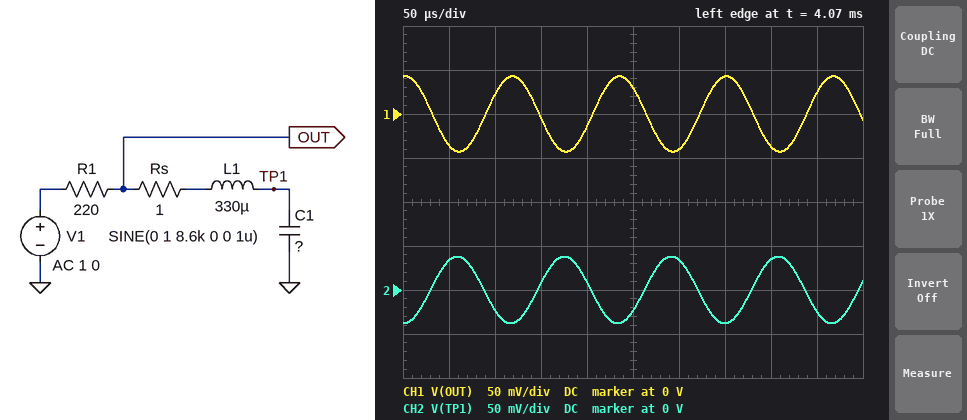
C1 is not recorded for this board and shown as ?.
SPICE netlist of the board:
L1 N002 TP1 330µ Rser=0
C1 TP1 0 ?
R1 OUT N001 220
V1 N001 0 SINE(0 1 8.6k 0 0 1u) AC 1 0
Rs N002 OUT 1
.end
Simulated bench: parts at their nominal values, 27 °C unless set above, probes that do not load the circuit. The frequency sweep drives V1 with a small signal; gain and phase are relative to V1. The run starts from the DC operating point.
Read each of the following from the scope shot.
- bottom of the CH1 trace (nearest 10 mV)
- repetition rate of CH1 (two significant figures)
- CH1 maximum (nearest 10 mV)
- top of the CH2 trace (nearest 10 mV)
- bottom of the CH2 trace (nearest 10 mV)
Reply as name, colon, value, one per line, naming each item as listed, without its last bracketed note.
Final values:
bottom of the CH1 trace: -40 mV
repetition rate of CH1: 8.6 kHz
CH1 maximum: 40 mV
top of the CH2 trace: 40 mV
bottom of the CH2 trace: -40 mV
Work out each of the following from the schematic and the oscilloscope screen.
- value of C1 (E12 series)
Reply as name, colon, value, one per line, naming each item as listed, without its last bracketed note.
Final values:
value of C1: 2.2 µF
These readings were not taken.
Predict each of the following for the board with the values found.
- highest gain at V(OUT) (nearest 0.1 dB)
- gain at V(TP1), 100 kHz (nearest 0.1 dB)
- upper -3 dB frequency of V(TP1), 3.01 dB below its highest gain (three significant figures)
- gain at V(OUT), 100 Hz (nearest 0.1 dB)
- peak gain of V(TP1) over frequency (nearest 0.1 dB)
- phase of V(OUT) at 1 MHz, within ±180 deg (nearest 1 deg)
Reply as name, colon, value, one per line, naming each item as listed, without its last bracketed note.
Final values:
highest gain at V(OUT): 0 dB
gain at V(TP1), 100 kHz: -52.4 dB
upper -3 dB frequency of V(TP1), 3.01 dB below its highest gain: 328 Hz
gain at V(OUT), 100 Hz: -0.4 dB
peak gain of V(TP1) over frequency: 0 dB
phase of V(OUT) at 1 MHz, within ±180 deg: 6 deg
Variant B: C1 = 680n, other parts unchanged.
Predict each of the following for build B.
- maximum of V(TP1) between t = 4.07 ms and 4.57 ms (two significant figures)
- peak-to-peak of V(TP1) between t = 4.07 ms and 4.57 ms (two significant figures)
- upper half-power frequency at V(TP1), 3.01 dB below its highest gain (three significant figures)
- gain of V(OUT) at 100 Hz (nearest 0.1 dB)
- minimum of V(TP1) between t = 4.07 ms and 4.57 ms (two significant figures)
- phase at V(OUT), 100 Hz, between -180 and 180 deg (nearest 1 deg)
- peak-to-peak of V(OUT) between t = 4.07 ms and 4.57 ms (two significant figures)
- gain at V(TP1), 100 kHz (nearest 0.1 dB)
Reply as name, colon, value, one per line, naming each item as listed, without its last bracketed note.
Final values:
maximum of V(TP1) between t = 4.07 ms and 4.57 ms: 120 mV
peak-to-peak of V(TP1) between t = 4.07 ms and 4.57 ms: 250 mV
upper half-power frequency at V(TP1), 3.01 dB below its highest gain: 1.07 kHz
gain of V(OUT) at 100 Hz: 0 dB
minimum of V(TP1) between t = 4.07 ms and 4.57 ms: -120 mV
phase at V(OUT), 100 Hz, between -180 and 180 deg: -5 deg
peak-to-peak of V(OUT) between t = 4.07 ms and 4.57 ms: 85 mV
gain at V(TP1), 100 kHz: -42.2 dB
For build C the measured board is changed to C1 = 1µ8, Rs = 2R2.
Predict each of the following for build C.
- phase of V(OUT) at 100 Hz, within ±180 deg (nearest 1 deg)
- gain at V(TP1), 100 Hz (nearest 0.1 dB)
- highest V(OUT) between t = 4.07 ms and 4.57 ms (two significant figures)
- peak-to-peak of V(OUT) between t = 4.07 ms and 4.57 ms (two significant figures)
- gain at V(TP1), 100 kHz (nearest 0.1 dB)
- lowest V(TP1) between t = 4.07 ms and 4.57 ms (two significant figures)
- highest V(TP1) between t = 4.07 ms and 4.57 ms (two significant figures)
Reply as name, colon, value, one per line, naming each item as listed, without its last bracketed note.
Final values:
phase of V(OUT) at 100 Hz, within ±180 deg: -14 deg
gain at V(TP1), 100 Hz: -0.3 dB
highest V(OUT) between t = 4.07 ms and 4.57 ms: 35 mV
peak-to-peak of V(OUT) between t = 4.07 ms and 4.57 ms: 71 mV
gain at V(TP1), 100 kHz: -50.7 dB
lowest V(TP1) between t = 4.07 ms and 4.57 ms: -46 mV
highest V(TP1) between t = 4.07 ms and 4.57 ms: 46 mV
